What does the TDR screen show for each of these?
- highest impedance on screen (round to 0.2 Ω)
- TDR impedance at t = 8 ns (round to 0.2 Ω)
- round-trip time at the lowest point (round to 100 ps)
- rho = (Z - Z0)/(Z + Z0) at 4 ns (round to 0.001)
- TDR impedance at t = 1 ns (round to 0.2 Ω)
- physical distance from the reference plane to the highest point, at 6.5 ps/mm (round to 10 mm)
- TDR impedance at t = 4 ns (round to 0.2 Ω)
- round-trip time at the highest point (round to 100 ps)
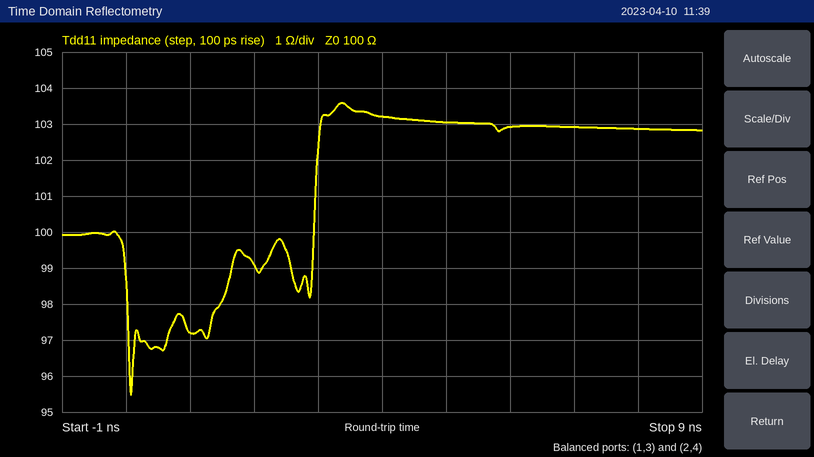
103.6 Ω
102.8 Ω
100 ps
+0.016
97.2 Ω
260 mm
103.2 Ω
3.4 ns
